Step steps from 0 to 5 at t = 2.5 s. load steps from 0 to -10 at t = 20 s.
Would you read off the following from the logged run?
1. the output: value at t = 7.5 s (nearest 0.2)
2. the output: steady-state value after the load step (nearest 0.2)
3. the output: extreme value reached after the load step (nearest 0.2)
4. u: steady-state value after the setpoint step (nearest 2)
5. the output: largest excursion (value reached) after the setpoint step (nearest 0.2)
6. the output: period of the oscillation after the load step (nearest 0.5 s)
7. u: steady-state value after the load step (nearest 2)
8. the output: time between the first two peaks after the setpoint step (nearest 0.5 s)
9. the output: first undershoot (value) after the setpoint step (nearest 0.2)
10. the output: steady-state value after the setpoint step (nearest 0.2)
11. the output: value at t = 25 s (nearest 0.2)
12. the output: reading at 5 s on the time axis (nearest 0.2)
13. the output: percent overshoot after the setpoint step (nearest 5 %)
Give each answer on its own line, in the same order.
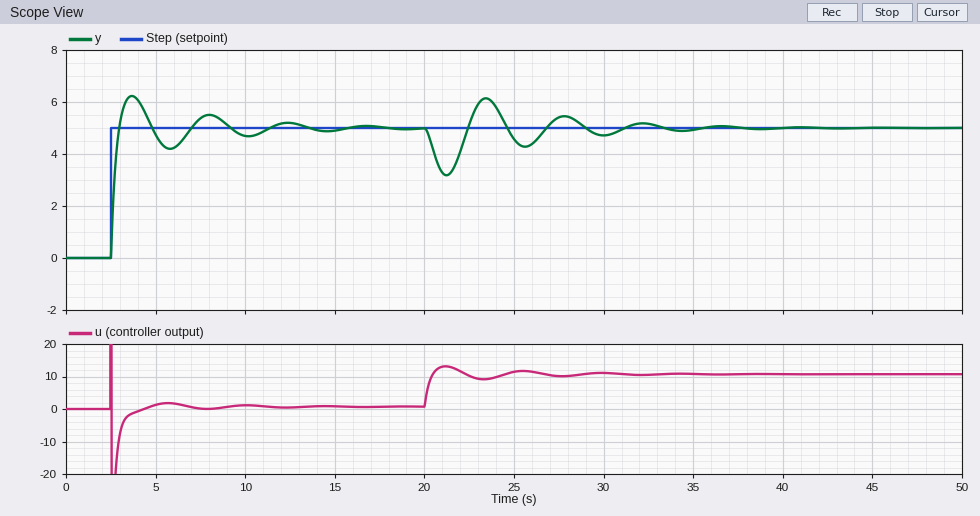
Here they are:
5.4
5.0
3.2
0
6.2
4.5 s
10
4.5 s
4.2
5.0
4.6
4.8
25 %
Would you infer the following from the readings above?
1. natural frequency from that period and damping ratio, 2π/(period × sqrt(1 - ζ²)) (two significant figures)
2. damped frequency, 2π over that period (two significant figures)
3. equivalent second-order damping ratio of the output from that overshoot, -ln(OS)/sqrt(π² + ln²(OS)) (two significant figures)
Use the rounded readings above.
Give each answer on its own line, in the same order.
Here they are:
1.5 rad/s
1.4 rad/s
0.40
